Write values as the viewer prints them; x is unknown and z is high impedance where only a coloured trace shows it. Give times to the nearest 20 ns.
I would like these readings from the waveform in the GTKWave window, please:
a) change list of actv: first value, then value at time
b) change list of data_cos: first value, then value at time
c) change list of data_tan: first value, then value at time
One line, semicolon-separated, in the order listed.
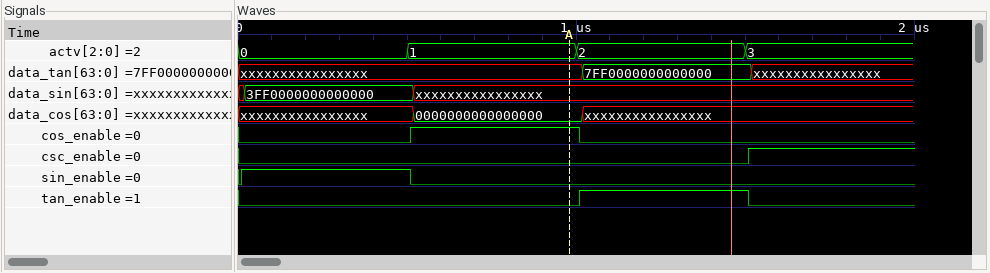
0, 1 at 500 ns, 2 at 1000 ns, 3 at 1500 ns; xxxxxxxxxxxxxxxx, 0000000000000000 at 520 ns, xxxxxxxxxxxxxxxx at 1020 ns; xxxxxxxxxxxxxxxx, 7FF0000000000000 at 1020 ns, xxxxxxxxxxxxxxxx at 1520 ns
